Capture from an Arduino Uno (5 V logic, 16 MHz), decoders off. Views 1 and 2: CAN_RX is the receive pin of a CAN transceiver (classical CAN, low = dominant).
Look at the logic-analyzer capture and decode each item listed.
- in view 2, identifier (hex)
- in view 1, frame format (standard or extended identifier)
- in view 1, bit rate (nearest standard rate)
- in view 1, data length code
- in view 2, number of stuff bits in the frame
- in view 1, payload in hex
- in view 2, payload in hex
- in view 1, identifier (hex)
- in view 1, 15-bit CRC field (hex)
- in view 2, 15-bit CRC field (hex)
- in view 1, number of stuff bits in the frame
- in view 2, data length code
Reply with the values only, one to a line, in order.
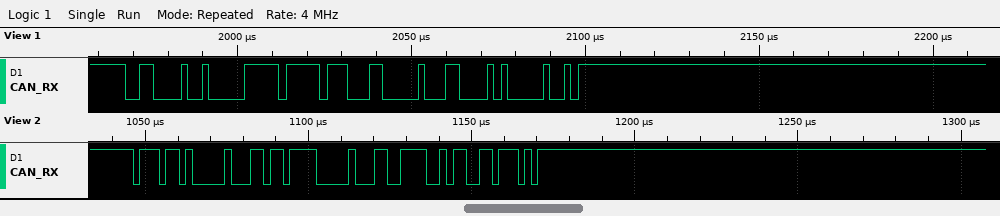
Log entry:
0x768
standard
500 kbit/s
3
2
FF C6 01
6F 00 CF
0x309
0x4280
0x166E
5
3
